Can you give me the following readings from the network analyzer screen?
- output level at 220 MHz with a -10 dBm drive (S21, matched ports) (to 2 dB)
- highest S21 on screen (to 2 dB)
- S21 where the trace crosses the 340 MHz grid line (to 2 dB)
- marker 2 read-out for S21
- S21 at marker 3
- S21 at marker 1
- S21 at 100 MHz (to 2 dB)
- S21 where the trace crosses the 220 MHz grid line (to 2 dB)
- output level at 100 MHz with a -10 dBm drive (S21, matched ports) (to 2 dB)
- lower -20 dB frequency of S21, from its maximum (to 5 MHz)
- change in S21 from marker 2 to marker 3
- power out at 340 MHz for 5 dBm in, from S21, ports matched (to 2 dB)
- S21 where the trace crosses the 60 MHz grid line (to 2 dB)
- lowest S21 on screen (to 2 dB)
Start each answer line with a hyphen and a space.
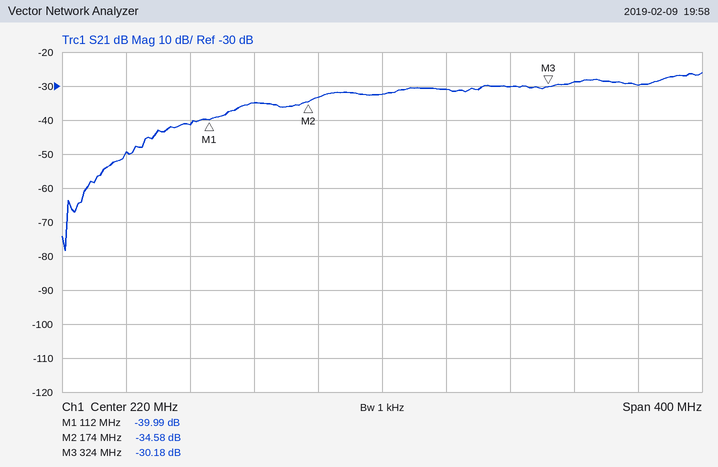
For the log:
- -42 dBm
- -26 dB
- -28 dB
- -34.58 dB
- -30.18 dB
- -39.99 dB
- -42 dB
- -32 dB
- -52 dBm
- 70 MHz
- 4.40 dB
- -24 dBm
- -50 dB
- -78 dB
